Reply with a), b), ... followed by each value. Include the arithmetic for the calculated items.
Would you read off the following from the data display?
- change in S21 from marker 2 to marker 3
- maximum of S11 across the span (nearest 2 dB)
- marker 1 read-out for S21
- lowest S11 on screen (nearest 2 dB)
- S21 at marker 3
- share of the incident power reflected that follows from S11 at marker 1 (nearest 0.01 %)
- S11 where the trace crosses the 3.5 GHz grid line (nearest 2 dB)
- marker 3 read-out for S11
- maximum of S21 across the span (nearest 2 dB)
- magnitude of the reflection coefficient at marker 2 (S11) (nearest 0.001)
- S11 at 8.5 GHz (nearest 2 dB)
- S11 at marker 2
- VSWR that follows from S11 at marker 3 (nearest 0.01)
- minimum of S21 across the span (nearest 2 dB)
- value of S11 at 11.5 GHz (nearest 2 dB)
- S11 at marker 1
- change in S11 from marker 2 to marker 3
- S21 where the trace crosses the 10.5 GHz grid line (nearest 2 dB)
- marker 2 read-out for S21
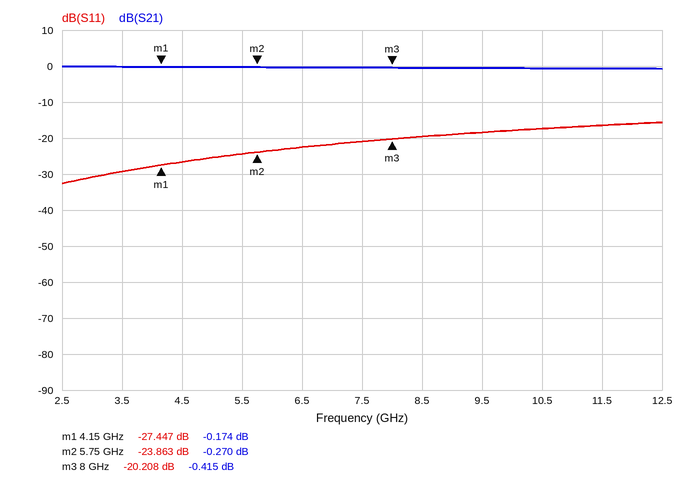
a) -0.415 − (-0.27) = -0.145 dB
b) -16 dB
c) -0.174 dB
d) -32 dB
e) -0.415 dB
f) 10^(-27.447/10) ≈ 0.18 %
g) -30 dB
h) -20.208 dB
i) 0 dB
j) 10^(-23.863/20) ≈ 0.064
k) -20 dB
l) -23.863 dB
m) (1 + 0.0976)/(1 − 0.0976) ≈ 1.22
n) 0 dB
o) -16 dB
p) -27.447 dB
q) -20.208 − (-23.863) = 3.655 dB
r) 0 dB
s) -0.270 dB
